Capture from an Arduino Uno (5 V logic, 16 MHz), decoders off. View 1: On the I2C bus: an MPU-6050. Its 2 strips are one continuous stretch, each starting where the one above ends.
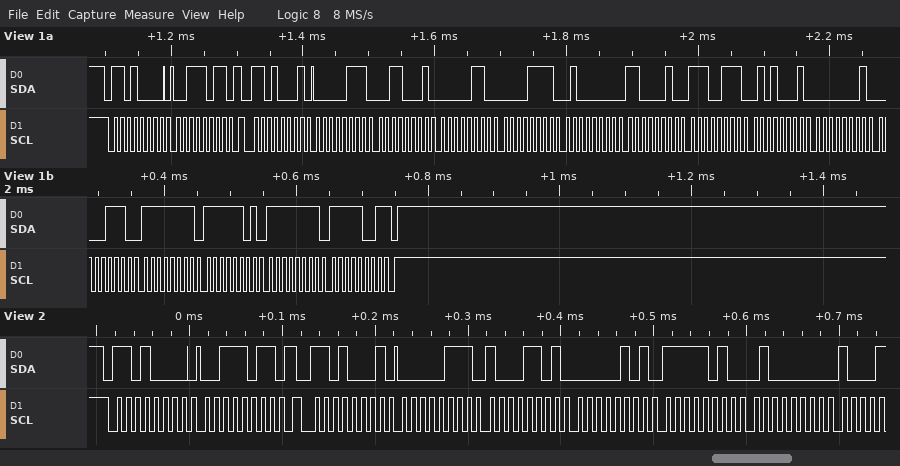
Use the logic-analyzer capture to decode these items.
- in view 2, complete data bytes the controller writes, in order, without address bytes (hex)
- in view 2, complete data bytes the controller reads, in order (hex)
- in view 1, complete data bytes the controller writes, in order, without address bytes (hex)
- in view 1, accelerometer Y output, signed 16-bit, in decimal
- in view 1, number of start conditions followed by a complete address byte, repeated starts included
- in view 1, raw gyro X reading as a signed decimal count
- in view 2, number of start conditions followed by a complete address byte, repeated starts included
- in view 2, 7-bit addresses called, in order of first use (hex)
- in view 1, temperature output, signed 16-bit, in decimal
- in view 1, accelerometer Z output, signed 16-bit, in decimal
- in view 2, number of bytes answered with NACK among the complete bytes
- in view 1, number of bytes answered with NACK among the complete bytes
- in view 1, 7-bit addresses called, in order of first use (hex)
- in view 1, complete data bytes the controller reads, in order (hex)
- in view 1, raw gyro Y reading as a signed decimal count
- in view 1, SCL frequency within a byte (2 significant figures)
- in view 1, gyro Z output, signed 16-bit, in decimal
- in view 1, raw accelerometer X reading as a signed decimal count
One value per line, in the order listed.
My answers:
3B
07 8D 05 FA 40
3B
1551
2
270
2
0x68
-6319
16578
0
1
0x68
07 31 06 0F 40 C2 E7 51 01 0E FF FD FF F9
-3
100 kHz
-7
1841
